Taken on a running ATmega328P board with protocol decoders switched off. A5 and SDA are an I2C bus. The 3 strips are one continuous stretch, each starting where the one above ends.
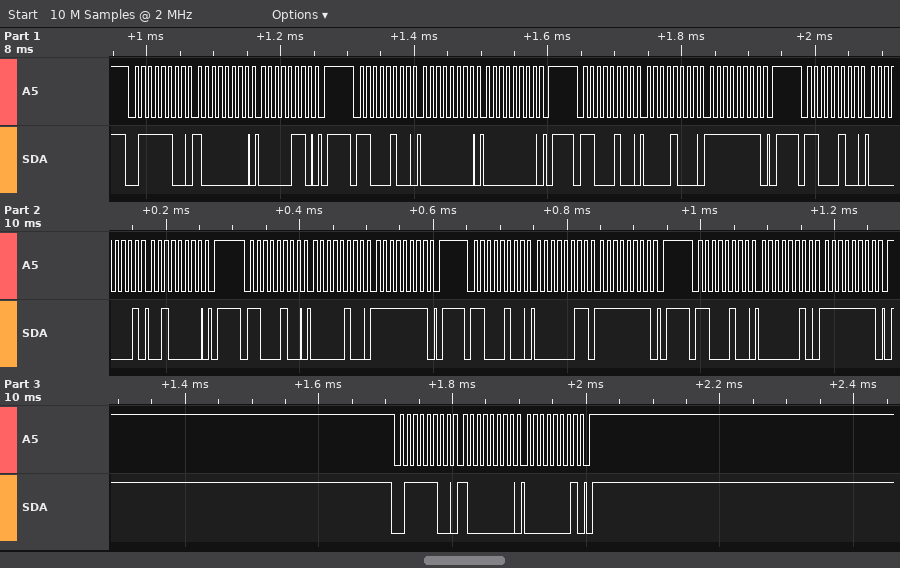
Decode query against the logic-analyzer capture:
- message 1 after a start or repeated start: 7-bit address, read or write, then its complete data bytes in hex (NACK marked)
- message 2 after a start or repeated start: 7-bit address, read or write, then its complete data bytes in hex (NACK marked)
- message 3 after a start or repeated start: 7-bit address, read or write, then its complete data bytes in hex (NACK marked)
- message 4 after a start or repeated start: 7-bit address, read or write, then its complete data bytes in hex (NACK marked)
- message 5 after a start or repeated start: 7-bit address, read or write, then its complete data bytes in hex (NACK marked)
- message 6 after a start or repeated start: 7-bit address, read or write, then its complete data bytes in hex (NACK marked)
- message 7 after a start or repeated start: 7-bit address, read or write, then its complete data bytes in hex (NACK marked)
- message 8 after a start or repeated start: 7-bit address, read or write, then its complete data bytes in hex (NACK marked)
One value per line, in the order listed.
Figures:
0x3E write: 80 06
0x62 write: 00 00
0x62 write: 08 FF
0x62 write: 01 20
0x62 write: 04 FF
0x62 write: 03 FF
0x62 write: 02 FF
0x3E write: 80 01
